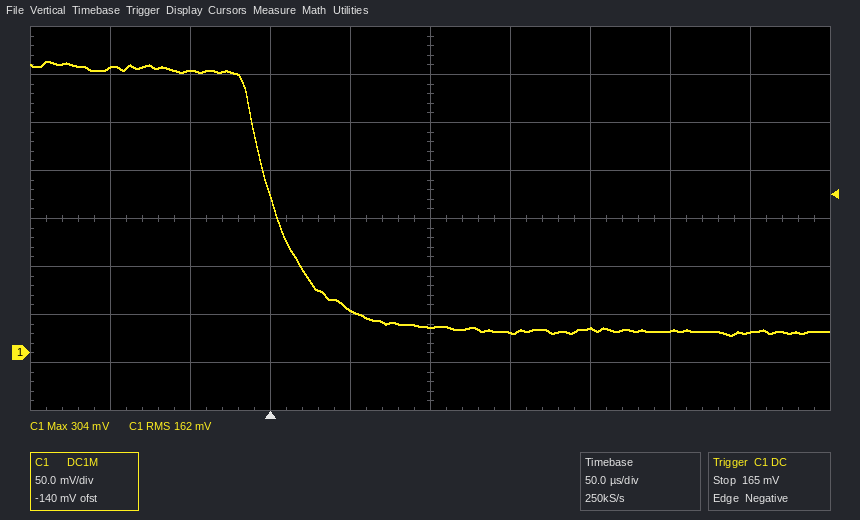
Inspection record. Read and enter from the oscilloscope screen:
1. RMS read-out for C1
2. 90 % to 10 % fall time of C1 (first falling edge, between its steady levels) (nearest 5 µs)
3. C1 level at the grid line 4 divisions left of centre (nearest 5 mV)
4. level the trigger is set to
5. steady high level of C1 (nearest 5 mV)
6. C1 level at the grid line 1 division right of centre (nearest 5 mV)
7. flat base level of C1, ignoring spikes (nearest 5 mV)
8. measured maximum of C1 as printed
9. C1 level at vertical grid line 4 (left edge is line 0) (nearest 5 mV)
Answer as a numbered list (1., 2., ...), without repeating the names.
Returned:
1. 162 mV
2. 60 µs
3. 295 mV
4. 165 mV
5. 295 mV
6. 20 mV
7. 20 mV
8. 304 mV
9. 45 mV
